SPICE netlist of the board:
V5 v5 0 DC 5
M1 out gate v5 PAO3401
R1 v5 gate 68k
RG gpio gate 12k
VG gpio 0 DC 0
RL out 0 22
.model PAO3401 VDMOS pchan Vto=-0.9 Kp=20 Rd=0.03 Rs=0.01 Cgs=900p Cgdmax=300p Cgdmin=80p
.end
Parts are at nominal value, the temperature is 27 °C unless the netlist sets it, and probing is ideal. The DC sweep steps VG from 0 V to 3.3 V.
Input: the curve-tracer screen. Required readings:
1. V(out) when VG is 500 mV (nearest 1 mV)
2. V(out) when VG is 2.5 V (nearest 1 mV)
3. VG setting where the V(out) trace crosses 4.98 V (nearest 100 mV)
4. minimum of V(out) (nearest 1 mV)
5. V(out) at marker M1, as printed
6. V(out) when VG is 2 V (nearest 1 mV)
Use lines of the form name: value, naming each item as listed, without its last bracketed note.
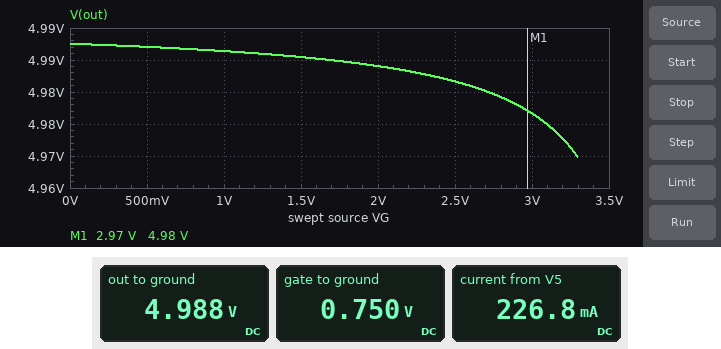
V(out) when VG is 500 mV: 4.987 V
V(out) when VG is 2.5 V: 4.982 V
VG setting where the V(out) trace crosses 4.98 V: 3.1 V
minimum of V(out): 4.970 V
V(out) at marker M1, as printed: 4.98 V
V(out) when VG is 2 V: 4.984 V
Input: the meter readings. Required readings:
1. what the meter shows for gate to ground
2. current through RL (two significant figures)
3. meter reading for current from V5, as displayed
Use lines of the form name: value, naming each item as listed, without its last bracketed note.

what the meter shows for gate to ground: 0.750 V
current through RL: 230 mA
meter reading for current from V5, as displayed: 226.8 mA
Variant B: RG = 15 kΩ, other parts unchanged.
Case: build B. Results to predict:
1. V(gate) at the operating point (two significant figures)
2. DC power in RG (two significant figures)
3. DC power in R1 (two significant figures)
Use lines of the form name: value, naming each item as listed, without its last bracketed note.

V(gate) at the operating point: 900 mV
DC power in RG: 54 µW
DC power in R1: 250 µW
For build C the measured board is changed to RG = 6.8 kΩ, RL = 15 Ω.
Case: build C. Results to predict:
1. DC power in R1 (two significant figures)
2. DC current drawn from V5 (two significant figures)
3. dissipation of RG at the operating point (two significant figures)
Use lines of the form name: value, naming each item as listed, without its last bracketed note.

DC power in R1: 300 µW
DC current drawn from V5: 330 mA
dissipation of RG at the operating point: 30 µW
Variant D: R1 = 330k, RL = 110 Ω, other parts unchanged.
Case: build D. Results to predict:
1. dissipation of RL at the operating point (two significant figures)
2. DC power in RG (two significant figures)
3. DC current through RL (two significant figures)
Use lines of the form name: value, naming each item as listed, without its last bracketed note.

dissipation of RL at the operating point: 230 mW
DC power in RG: 2.6 µW
DC current through RL: 45 mA
